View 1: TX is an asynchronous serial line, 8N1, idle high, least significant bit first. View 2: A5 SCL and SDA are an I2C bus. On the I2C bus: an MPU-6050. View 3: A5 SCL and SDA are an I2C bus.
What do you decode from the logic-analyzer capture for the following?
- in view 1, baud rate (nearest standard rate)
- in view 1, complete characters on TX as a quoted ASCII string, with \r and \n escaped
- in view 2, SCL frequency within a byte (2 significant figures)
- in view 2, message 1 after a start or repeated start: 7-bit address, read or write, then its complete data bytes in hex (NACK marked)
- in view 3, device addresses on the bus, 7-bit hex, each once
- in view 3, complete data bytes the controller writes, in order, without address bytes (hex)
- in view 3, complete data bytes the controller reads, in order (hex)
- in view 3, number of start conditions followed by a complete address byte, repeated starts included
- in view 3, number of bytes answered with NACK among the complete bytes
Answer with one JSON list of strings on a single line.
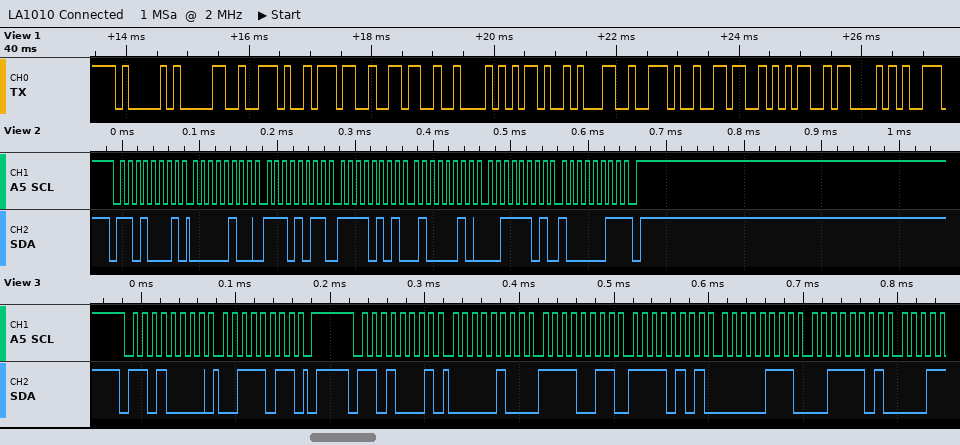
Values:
["9600 baud", "\"A0.76B-1.65C\"", "100 kHz", "0x68 read: 04 EB F5 42 3D 83 NACK", "0x68", "3B", "04 F3 F5 07 3D", "2", "0"]
